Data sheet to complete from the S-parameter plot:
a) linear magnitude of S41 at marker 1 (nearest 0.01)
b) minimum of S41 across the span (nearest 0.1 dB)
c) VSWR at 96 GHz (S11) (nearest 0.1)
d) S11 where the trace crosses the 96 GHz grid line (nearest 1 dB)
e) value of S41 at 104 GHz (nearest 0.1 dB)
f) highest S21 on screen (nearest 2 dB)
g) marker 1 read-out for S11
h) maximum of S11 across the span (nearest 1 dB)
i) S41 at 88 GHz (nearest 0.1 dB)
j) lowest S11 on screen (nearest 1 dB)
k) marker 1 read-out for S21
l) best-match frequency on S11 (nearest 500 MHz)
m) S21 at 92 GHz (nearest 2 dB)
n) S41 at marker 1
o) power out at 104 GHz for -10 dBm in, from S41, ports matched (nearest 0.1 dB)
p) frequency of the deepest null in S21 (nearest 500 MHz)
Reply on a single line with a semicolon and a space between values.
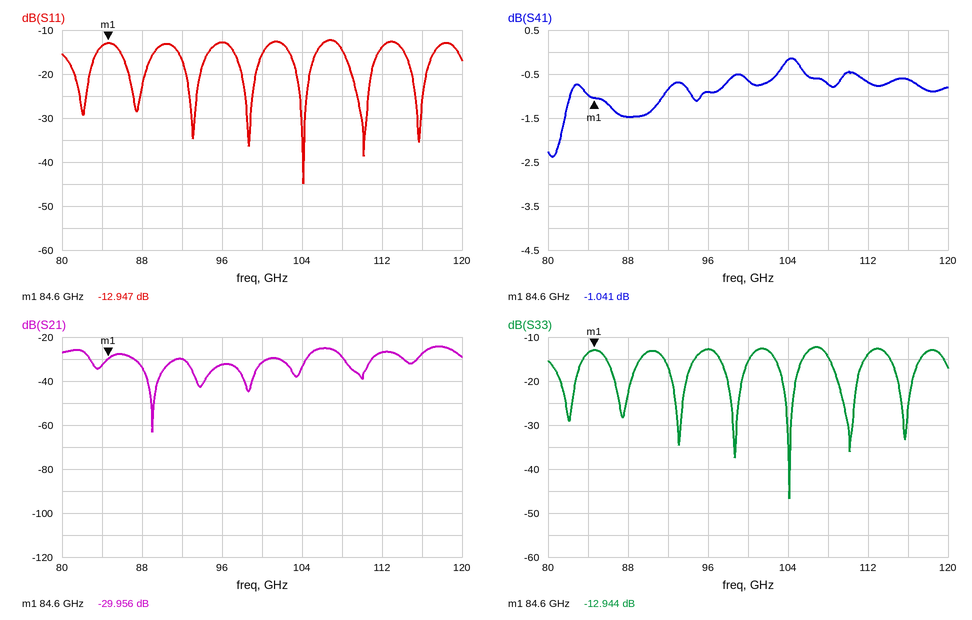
0.89; -2.4 dB; 1.6; -13 dB; -0.2 dB; -24 dB; -12.947 dB; -12 dB; -1.5 dB; -45 dB; -29.956 dB; 104.0 GHz; -30 dB; -1.041 dB; -10.2 dBm; 89.0 GHz
